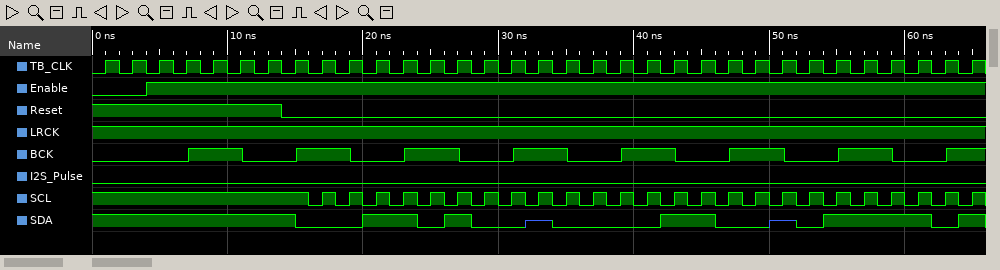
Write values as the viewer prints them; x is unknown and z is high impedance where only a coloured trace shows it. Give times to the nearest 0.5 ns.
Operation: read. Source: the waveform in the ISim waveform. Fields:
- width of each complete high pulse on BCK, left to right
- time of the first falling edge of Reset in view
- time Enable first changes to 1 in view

4 ns, 4 ns, 4 ns, 4 ns, 4 ns, 4 ns, 4 ns
14 ns
4 ns
